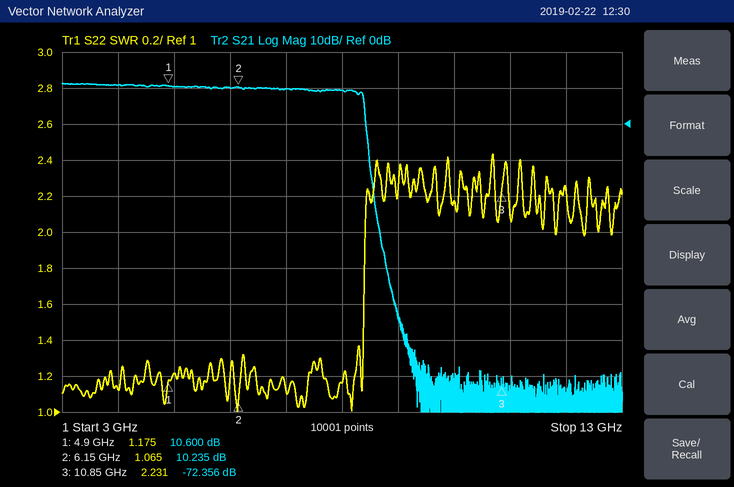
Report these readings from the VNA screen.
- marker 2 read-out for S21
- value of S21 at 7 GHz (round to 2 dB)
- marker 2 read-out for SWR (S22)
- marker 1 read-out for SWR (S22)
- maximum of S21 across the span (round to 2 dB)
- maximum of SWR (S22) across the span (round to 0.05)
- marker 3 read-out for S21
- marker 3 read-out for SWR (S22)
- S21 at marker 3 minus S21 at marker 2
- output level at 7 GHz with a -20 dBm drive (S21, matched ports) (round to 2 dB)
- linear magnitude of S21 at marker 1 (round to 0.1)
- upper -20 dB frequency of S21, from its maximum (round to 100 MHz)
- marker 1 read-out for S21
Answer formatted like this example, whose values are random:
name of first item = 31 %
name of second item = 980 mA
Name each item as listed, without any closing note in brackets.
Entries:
marker 2 read-out for S21 = 10.235 dB
value of S21 at 7 GHz = 10 dB
marker 2 read-out for SWR = 1.065
marker 1 read-out for SWR = 1.175
maximum of S21 across the span = 12 dB
maximum of SWR (S22) across the span = 2.45
marker 3 read-out for S21 = -72.356 dB
marker 3 read-out for SWR = 2.231
S21 at marker 3 minus S21 at marker 2 = -82.591 dB
output level at 7 GHz with a -20 dBm drive (S21, matched ports) = -10 dBm
linear magnitude of S21 at marker 1 = 3.4
upper -20 dB frequency of S21, from its maximum = 8.5 GHz
marker 1 read-out for S21 = 10.600 dB
